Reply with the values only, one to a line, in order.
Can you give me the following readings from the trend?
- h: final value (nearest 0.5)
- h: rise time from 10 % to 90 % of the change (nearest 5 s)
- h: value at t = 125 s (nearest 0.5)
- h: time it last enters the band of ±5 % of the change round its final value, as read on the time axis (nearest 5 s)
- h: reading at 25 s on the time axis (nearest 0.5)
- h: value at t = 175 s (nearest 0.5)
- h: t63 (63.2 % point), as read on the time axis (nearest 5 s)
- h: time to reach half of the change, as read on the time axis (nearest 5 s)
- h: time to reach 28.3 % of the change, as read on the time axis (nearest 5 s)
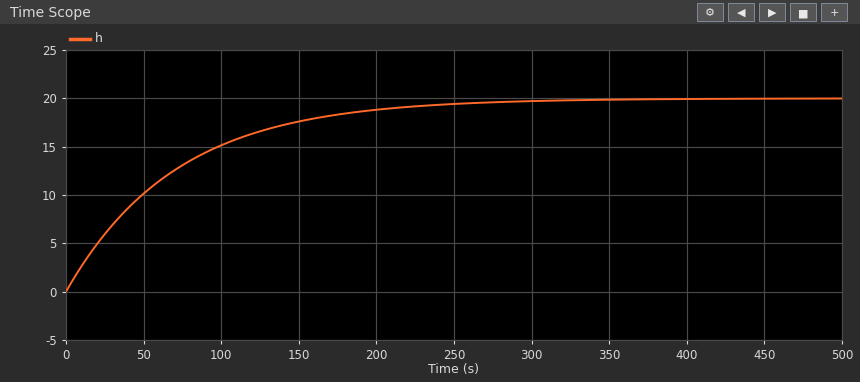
20.0
155 s
16.5
210 s
6.0
18.5
70 s
50 s
25 s
